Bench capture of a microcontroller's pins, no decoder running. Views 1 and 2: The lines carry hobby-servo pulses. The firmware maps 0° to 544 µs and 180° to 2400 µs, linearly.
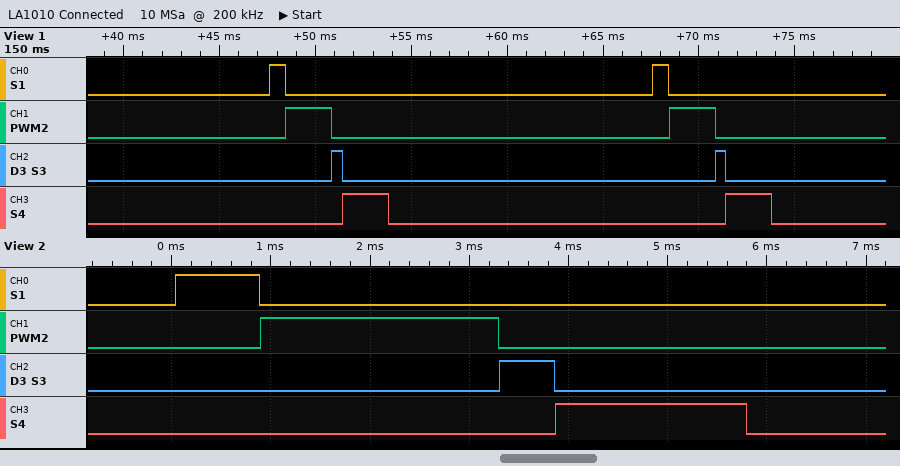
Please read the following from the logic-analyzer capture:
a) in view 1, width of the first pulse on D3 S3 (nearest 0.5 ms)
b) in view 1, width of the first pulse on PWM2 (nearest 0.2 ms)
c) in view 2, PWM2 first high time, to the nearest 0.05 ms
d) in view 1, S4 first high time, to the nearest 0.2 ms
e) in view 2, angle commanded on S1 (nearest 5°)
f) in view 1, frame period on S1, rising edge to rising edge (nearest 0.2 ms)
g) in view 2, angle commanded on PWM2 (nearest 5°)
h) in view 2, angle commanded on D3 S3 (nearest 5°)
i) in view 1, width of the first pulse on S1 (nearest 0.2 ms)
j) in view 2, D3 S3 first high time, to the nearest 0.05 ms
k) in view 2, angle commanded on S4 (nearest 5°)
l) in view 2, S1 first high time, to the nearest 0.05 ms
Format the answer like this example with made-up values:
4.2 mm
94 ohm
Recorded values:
0.5 ms
2.4 ms
2.40 ms
2.4 ms
30°
20.0 ms
180°
0°
0.8 ms
0.55 ms
135°
0.85 ms
